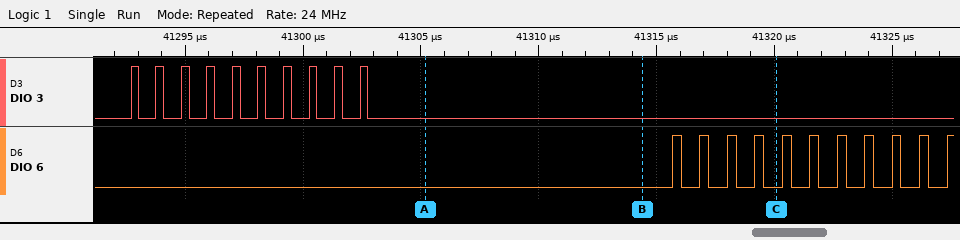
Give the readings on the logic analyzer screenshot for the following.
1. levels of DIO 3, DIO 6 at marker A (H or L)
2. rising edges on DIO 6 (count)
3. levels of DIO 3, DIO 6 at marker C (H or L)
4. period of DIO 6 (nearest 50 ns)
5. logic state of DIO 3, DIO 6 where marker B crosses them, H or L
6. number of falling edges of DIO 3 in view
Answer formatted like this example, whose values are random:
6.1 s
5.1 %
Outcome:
DIO 3=L, DIO 6=L
11
DIO 3=L, DIO 6=L
1150 ns
DIO 3=L, DIO 6=L
10
